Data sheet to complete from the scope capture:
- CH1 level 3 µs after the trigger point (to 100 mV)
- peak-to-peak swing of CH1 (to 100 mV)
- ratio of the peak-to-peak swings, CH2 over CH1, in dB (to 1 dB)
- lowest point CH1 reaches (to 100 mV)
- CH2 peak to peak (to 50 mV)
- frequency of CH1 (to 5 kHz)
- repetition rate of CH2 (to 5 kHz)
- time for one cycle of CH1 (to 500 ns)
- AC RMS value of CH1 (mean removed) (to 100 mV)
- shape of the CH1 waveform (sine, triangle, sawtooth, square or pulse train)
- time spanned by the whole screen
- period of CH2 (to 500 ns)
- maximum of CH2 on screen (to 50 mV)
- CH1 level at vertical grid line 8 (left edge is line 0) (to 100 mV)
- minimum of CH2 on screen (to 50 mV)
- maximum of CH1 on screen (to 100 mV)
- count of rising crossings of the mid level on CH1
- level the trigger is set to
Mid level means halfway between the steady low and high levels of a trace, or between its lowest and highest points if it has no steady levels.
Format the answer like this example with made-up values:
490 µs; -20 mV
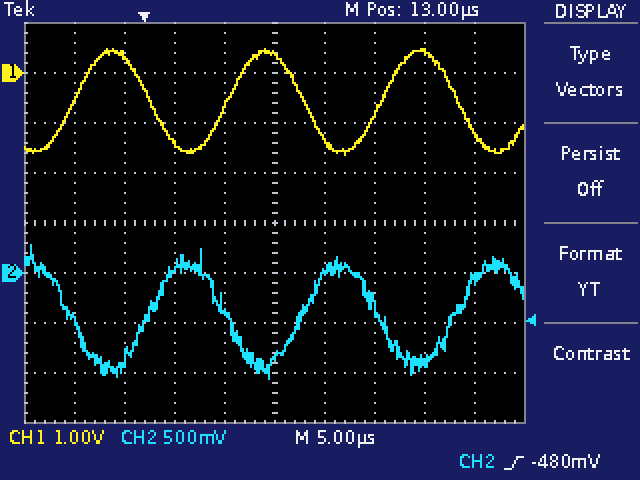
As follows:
-1.4 V; 2.1 V; -4 dB; -1.6 V; 1.35 V; 65 kHz; 65 kHz; 15.5 µs; 700 mV; sine; 50 µs; 15.5 µs; 300 mV; 400 mV; -1.05 V; 500 mV; 3; -480 mV
